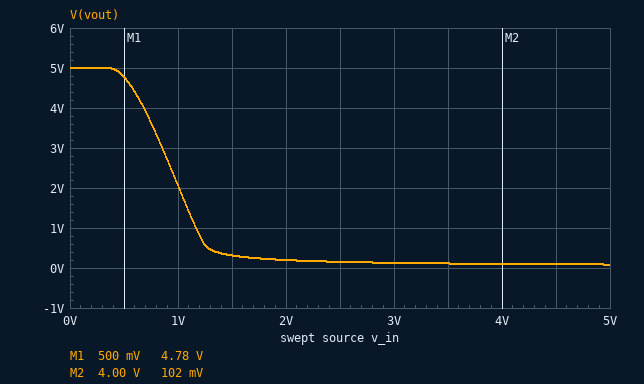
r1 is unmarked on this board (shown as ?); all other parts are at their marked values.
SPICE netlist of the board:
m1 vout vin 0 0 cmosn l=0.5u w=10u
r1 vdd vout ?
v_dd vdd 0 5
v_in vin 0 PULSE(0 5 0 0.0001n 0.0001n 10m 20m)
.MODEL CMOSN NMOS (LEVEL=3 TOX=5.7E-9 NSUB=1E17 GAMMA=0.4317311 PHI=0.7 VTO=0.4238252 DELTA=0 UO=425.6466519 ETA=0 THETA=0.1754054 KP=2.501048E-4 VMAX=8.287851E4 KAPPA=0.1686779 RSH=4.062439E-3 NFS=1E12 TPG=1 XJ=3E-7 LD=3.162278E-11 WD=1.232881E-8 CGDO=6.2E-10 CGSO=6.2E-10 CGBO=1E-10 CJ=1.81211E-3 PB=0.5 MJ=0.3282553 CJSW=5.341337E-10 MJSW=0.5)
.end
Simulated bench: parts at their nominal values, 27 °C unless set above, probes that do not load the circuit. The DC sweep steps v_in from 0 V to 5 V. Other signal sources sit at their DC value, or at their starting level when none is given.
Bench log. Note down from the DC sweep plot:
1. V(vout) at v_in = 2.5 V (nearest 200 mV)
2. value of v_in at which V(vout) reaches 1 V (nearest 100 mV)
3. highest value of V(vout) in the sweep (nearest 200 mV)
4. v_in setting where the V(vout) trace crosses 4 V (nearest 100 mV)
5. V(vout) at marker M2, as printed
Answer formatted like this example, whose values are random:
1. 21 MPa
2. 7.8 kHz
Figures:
1. 200 mV
2. 1.2 V
3. 5.0 V
4. 700 mV
5. 102 mV
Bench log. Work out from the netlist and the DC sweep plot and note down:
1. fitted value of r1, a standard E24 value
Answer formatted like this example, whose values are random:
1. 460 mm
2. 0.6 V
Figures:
1. 4.7 kΩ
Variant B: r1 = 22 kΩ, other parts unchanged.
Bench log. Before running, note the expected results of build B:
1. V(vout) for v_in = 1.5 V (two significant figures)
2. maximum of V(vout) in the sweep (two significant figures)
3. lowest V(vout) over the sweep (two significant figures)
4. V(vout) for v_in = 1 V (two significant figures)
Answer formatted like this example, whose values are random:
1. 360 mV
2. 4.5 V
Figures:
1. 51 mV
2. 5.0 V
3. 18 mV
4. 91 mV
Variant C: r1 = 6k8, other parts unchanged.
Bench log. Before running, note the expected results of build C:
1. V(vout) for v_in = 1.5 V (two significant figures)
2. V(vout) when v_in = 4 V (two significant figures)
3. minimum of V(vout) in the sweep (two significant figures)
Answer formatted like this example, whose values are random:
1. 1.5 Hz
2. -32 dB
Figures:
1. 190 mV
2. 69 mV
3. 59 mV
